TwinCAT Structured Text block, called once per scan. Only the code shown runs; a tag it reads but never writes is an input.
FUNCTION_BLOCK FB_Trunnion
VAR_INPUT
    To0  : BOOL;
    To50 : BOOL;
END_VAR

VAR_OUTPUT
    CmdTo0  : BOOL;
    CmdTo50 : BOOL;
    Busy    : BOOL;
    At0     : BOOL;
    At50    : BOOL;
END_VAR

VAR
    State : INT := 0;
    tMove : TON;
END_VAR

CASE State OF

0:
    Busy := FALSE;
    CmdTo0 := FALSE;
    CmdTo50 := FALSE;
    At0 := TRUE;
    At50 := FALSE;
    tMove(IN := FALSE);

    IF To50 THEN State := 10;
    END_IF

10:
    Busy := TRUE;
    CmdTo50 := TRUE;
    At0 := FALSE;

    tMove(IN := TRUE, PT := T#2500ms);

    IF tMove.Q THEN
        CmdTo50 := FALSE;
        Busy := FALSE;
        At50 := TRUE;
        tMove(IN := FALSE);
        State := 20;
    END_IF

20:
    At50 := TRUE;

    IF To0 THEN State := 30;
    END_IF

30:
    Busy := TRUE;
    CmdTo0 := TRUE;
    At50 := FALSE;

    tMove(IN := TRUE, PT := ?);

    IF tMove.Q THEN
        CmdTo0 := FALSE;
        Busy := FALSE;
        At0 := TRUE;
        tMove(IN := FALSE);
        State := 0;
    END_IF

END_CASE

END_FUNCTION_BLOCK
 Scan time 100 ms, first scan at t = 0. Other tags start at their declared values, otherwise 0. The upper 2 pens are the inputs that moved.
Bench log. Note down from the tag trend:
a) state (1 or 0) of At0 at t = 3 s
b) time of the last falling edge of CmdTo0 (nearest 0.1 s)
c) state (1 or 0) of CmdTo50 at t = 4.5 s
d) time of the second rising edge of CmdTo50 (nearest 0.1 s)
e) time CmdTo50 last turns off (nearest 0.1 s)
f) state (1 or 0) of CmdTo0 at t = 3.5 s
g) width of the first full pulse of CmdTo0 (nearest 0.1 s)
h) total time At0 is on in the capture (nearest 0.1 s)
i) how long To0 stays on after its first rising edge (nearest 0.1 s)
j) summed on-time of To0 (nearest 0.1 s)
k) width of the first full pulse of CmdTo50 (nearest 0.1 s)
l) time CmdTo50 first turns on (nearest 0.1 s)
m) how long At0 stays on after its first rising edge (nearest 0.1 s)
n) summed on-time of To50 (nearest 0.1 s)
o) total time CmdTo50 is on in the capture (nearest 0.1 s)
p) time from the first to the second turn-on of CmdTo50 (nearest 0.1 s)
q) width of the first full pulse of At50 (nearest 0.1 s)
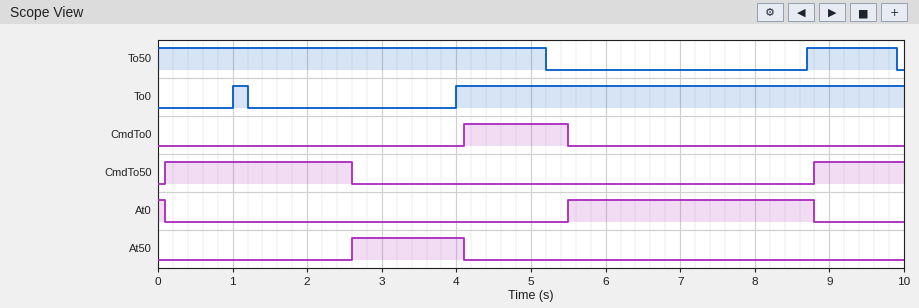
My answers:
0
5.5 s
0
8.8 s
2.6 s
0
1.4 s
3.4 s
0.2 s
6.2 s
2.5 s
0.1 s
3.3 s
6.4 s
3.7 s
8.7 s
1.5 s
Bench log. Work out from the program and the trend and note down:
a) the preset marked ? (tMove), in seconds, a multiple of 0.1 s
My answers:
1.4 s
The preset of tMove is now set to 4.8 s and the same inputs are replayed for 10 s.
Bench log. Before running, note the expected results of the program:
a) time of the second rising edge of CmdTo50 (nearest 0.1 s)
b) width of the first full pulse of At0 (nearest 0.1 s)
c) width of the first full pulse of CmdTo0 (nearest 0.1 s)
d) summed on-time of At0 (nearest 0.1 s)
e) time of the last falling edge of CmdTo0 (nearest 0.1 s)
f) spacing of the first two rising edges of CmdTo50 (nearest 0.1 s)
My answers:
9.1 s
0.2 s
4.8 s
0.3 s
8.9 s
9.0 s
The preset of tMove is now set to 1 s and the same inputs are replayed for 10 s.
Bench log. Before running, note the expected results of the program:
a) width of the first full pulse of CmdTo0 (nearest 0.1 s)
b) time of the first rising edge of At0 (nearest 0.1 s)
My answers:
1.0 s
5.1 s
